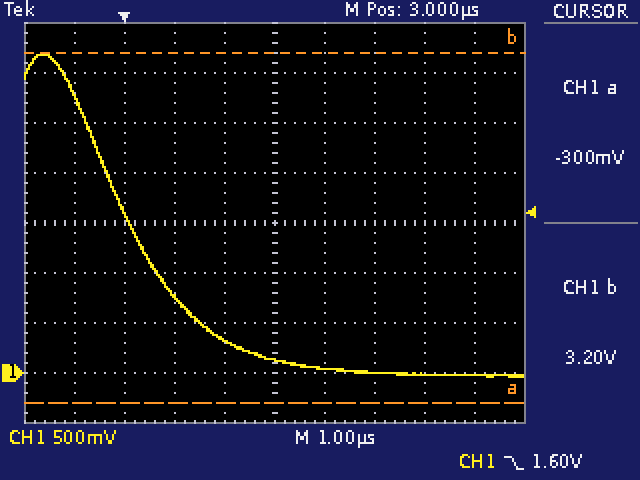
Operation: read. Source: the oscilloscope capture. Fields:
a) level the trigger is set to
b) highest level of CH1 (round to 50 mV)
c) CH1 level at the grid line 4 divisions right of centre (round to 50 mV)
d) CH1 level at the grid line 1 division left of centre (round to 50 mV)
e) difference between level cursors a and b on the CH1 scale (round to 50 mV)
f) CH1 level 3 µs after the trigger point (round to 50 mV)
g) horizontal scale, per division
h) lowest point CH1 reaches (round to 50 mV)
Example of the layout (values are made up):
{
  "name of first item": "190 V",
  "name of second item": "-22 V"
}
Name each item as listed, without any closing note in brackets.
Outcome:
{
  "level the trigger is set to": "1.60 V",
  "highest level of CH1": "3.20 V",
  "CH1 level at the grid line 4 divisions right of centre": "0 mV",
  "CH1 level at the grid line 1 division left of centre": "350 mV",
  "difference between level cursors a and b on the CH1 scale": "3.50 V",
  "CH1 level 3 µs after the trigger point": "150 mV",
  "horizontal scale, per division": "1 µs",
  "lowest point CH1 reaches": "-50 mV"
}
